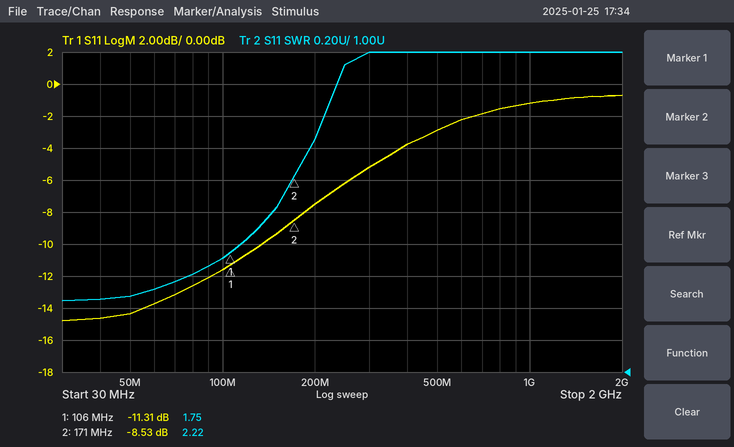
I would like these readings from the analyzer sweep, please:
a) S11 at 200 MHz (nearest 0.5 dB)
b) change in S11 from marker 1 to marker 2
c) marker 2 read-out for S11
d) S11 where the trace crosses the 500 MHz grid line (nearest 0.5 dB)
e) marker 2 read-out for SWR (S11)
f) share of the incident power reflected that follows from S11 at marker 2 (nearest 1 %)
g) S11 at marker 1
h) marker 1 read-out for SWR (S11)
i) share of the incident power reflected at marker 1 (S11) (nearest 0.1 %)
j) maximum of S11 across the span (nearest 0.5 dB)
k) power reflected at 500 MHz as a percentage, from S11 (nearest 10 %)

-7.5 dB
2.78 dB
-8.53 dB
-3.0 dB
2.22
14 %
-11.31 dB
1.75
7.4 %
-0.5 dB
50 %
